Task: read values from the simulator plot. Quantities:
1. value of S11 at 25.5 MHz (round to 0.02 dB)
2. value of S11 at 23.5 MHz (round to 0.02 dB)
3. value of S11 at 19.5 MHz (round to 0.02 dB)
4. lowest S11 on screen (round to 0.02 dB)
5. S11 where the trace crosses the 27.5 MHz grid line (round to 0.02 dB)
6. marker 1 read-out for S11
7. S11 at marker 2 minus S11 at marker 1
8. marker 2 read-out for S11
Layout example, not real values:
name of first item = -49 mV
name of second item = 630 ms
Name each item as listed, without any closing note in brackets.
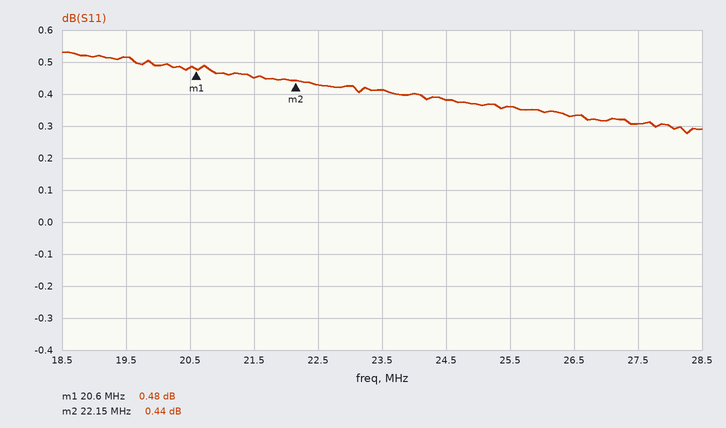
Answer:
value of S11 at 25.5 MHz = 0.36 dB
value of S11 at 23.5 MHz = 0.42 dB
value of S11 at 19.5 MHz = 0.52 dB
lowest S11 on screen = 0.28 dB
S11 where the trace crosses the 27.5 MHz grid line = 0.30 dB
marker 1 read-out for S11 = 0.48 dB
S11 at marker 2 minus S11 at marker 1 = -0.04 dB
marker 2 read-out for S11 = 0.44 dB
